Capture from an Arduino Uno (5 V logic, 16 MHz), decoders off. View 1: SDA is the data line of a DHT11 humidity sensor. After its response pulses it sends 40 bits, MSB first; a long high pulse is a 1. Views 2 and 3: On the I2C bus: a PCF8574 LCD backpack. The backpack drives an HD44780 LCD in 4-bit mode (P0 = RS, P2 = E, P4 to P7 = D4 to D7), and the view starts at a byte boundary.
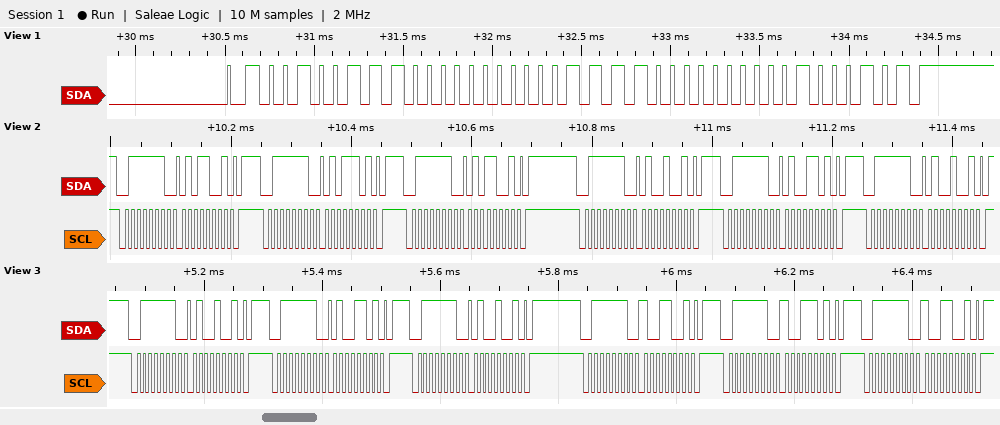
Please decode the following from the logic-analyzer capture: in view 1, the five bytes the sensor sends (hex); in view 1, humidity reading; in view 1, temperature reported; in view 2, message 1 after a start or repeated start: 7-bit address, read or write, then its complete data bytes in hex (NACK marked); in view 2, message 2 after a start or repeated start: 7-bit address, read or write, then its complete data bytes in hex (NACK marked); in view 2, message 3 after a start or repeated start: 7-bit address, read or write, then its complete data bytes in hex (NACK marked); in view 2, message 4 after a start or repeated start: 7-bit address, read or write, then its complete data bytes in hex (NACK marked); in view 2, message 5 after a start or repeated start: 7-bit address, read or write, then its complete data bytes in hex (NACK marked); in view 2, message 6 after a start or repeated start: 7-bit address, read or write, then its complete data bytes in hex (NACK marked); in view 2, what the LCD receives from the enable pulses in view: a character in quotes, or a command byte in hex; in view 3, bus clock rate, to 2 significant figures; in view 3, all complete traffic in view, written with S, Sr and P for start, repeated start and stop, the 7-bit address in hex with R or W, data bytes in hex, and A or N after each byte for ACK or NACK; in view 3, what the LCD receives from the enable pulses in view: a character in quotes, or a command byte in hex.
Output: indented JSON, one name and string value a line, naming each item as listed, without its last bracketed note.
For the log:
{
  "in view 1, the five bytes the sensor sends": "27 00 1E 00 45",
  "in view 1, humidity reading": "39 %",
  "in view 1, temperature reported": "30.0 °C",
  "in view 2, message 1 after a start or repeated start: 7-bit address, read or write, then its complete data bytes in hex": "0x3F write: 59",
  "in view 2, message 2 after a start or repeated start: 7-bit address, read or write, then its complete data bytes in hex": "0x3F write: 5D",
  "in view 2, message 3 after a start or repeated start: 7-bit address, read or write, then its complete data bytes in hex": "0x3F write: 59",
  "in view 2, message 4 after a start or repeated start: 7-bit address, read or write, then its complete data bytes in hex": "0x3F write: 49",
  "in view 2, message 5 after a start or repeated start: 7-bit address, read or write, then its complete data bytes in hex": "0x3F write: 4D",
  "in view 2, message 6 after a start or repeated start: 7-bit address, read or write, then its complete data bytes in hex": "0x3F write: 49",
  "in view 2, what the LCD receives from the enable pulses in view: a character in quotes, or a command byte in hex": "'T'",
  "in view 3, bus clock rate, to 2 significant figures": "100 kHz",
  "in view 3, all complete traffic in view, written with S, Sr and P for start, repeated start and stop, the 7-bit address in hex with R or W, data bytes in hex, and A or N after each byte for ACK or NACK": "S 3FW A 49 A P S 3FW A 4D A P S 3FW A 49 A P S 3FW A 99 A P S 3FW A 9D A P S 3FW A 99 A P",
  "in view 3, what the LCD receives from the enable pulses in view: a character in quotes, or a command byte in hex": "'I'"
}
